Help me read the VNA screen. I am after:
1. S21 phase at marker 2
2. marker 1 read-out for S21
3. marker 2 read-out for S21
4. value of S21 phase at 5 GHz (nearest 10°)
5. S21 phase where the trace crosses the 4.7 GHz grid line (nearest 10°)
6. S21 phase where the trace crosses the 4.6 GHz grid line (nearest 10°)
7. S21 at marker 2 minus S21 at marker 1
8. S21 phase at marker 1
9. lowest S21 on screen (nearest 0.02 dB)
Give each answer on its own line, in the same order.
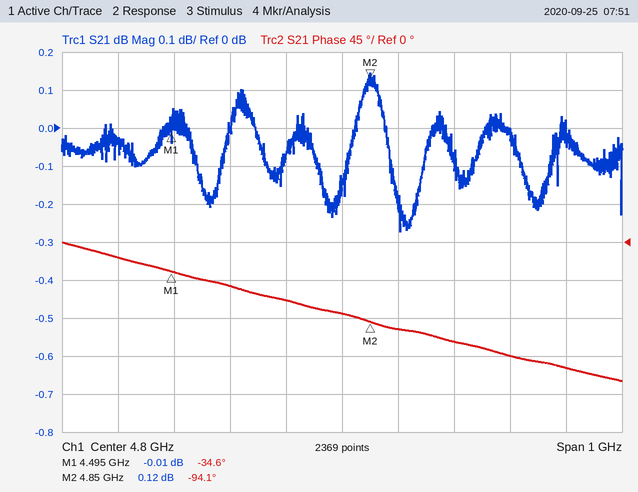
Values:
-94.1°
-0.01 dB
0.12 dB
-120°
-70°
-50°
0.13 dB
-34.6°
-0.28 dB
